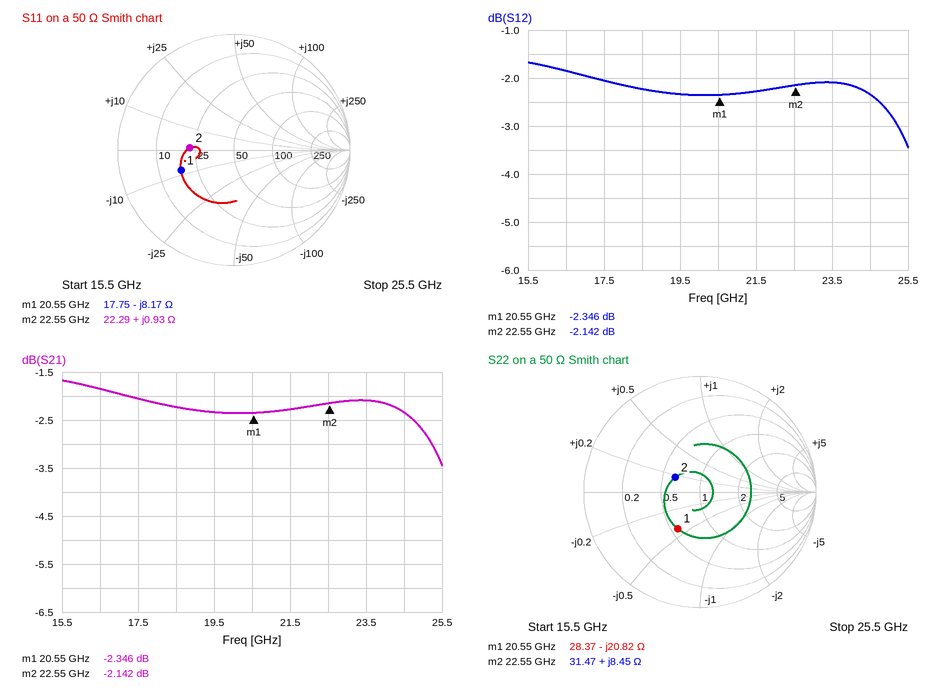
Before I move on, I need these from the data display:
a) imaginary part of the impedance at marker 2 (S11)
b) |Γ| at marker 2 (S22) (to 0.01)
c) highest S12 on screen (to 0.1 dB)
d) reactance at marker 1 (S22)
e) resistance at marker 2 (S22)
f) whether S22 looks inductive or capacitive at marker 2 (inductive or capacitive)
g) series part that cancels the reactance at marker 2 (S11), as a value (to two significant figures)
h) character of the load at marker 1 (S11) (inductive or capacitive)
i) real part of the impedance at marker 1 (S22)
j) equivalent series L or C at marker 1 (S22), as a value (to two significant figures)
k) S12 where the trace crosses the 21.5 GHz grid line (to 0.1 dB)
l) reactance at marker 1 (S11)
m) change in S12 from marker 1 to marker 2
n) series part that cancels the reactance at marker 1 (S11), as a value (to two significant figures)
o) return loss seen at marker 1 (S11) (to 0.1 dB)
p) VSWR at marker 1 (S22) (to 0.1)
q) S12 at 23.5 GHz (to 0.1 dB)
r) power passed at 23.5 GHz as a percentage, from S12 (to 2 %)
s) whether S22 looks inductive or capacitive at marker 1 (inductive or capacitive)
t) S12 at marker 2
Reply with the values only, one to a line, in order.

+0.93 Ω
0.25
-1.7 dB
-20.82 Ω
31.47 Ω
inductive
7.6 pF
capacitive
28.37 Ω
370 fF
-2.3 dB
-8.17 Ω
0.204 dB
63 pH
6.2 dB
2.2
-2.1 dB
62 %
capacitive
-2.142 dB
